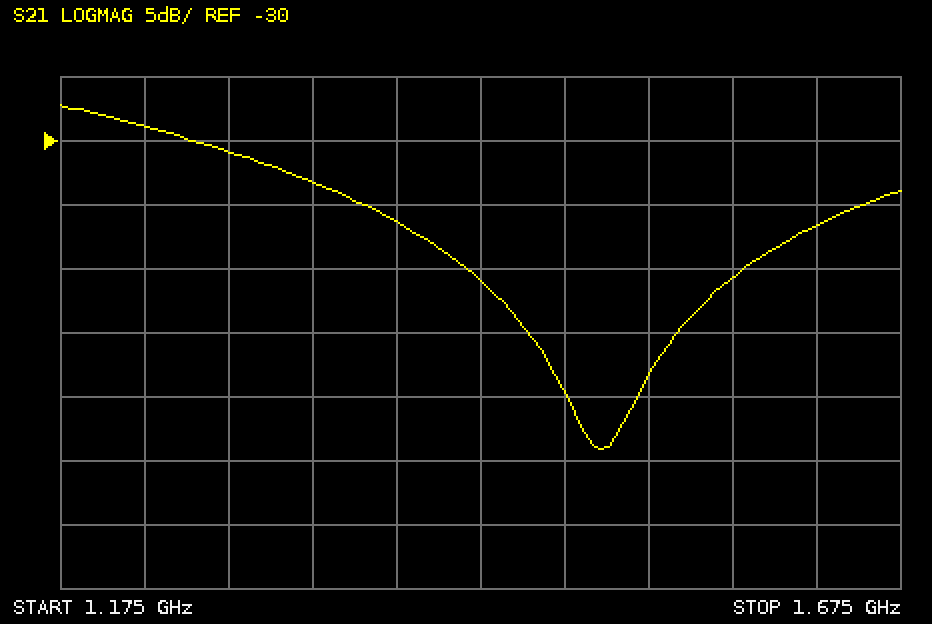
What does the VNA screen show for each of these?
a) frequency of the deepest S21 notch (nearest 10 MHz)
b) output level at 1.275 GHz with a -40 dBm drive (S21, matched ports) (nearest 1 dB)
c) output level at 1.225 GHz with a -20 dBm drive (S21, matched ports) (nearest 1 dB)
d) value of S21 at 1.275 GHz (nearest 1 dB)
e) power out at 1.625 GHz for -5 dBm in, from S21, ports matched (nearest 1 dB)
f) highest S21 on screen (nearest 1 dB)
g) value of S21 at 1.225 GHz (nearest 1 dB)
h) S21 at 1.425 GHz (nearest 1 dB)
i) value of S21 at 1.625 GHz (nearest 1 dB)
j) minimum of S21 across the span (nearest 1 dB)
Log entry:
1.50 GHz
-71 dBm
-49 dBm
-31 dB
-42 dBm
-27 dB
-29 dB
-41 dB
-37 dB
-54 dB
